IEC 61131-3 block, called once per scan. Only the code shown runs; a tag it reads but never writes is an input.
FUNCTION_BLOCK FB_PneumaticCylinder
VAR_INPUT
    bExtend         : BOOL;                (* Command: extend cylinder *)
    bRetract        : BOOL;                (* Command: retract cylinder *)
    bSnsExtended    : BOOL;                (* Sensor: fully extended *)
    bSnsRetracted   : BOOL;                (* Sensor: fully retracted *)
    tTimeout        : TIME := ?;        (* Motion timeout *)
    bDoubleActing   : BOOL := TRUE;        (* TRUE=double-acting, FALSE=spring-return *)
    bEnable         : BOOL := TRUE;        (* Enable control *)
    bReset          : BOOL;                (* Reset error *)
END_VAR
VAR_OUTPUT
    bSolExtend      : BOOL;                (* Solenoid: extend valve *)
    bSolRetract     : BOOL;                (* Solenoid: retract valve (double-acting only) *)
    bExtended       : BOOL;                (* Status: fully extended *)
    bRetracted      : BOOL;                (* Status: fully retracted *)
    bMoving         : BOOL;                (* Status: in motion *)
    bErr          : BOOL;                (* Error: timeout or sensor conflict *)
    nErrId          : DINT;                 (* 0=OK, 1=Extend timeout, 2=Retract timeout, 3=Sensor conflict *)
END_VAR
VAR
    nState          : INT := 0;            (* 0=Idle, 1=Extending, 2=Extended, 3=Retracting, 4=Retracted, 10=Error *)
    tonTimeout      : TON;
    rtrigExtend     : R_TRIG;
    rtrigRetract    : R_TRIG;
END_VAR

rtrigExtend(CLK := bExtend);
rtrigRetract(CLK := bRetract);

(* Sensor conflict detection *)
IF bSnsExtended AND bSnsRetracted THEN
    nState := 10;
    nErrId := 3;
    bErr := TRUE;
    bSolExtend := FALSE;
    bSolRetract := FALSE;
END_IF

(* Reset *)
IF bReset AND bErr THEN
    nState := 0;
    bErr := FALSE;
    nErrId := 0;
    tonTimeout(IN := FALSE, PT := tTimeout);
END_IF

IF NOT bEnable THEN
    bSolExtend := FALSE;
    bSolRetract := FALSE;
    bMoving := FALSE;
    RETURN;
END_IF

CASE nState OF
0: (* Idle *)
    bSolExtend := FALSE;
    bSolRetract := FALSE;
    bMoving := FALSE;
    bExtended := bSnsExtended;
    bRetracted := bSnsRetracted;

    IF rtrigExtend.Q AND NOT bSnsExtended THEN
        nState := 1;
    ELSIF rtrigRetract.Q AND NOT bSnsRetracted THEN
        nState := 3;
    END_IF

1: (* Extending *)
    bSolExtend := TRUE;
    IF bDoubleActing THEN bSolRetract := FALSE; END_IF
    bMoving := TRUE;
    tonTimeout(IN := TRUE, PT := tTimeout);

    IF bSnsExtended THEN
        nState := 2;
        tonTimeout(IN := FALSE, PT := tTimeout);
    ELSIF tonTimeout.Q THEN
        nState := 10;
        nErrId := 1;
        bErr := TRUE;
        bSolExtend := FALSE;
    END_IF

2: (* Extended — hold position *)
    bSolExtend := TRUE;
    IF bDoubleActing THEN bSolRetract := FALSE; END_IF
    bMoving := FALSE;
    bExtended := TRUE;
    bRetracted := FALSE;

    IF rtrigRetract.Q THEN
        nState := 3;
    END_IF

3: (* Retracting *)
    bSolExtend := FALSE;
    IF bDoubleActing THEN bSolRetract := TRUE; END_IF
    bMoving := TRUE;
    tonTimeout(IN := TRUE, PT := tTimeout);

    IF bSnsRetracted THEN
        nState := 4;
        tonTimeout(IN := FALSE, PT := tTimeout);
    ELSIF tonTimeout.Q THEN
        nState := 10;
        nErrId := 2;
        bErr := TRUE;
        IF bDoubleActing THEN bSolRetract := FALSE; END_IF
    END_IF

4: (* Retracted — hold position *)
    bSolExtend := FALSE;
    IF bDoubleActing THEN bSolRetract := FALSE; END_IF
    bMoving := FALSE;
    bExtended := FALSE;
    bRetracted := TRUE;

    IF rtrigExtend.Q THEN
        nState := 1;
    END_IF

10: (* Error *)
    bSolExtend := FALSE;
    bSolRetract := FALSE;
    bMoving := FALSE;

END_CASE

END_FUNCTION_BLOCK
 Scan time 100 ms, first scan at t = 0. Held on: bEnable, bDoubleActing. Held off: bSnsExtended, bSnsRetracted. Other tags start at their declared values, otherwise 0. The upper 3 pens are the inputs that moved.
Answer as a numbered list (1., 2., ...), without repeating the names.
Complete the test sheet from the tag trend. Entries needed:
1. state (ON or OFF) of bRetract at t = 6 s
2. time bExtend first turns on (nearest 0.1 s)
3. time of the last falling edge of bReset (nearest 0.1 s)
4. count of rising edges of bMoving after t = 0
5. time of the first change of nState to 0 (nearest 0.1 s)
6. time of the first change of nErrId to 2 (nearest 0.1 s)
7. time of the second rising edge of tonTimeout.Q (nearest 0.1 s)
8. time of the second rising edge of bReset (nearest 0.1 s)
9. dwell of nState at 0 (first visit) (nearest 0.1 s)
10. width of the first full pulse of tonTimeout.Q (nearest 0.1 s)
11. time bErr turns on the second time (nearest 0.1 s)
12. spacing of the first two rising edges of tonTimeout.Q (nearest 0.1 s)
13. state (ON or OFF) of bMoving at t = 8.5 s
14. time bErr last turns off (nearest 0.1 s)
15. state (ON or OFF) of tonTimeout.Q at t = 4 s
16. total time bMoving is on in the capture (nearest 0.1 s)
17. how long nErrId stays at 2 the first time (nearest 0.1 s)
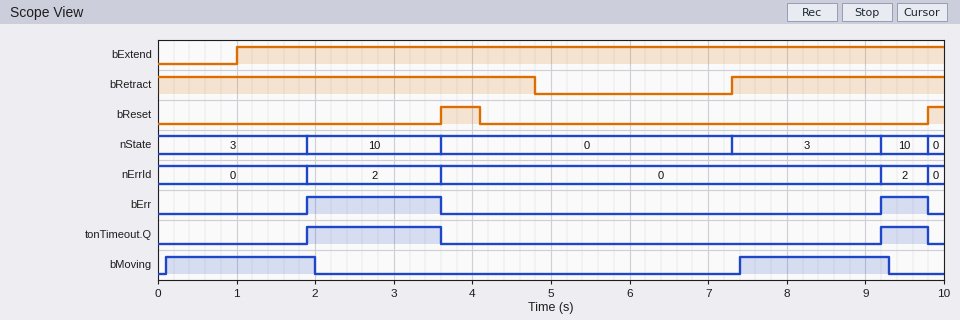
1. OFF
2. 1.0 s
3. 4.1 s
4. 2
5. 3.6 s
6. 1.9 s
7. 9.2 s
8. 9.8 s
9. 3.7 s
10. 1.7 s
11. 9.2 s
12. 7.3 s
13. ON
14. 9.8 s
15. OFF
16. 3.8 s
17. 1.7 s
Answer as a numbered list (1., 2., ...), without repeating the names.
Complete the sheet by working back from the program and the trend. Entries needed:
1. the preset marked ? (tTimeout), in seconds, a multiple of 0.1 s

1. 1.8 s
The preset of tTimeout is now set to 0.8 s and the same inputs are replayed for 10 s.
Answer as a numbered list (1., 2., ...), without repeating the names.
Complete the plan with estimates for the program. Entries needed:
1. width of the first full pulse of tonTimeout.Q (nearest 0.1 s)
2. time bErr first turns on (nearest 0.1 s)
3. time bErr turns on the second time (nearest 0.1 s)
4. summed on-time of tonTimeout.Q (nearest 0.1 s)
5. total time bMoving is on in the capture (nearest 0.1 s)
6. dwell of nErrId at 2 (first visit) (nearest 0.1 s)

1. 2.7 s
2. 0.9 s
3. 8.2 s
4. 4.3 s
5. 1.8 s
6. 2.7 s
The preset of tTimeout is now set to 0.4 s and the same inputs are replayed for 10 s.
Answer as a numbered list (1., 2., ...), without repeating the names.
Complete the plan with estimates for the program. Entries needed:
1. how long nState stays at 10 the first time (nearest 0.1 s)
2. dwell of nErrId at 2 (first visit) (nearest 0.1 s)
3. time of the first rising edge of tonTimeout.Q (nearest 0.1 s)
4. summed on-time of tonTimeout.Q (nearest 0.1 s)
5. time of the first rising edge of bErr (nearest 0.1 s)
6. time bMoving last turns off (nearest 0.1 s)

1. 3.1 s
2. 3.1 s
3. 0.5 s
4. 5.1 s
5. 0.5 s
6. 7.9 s
